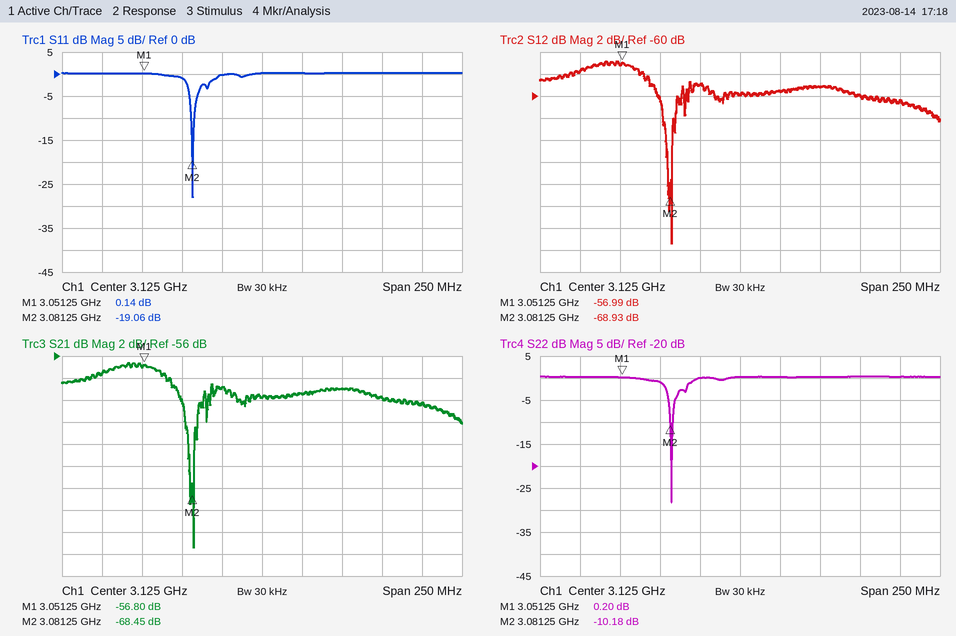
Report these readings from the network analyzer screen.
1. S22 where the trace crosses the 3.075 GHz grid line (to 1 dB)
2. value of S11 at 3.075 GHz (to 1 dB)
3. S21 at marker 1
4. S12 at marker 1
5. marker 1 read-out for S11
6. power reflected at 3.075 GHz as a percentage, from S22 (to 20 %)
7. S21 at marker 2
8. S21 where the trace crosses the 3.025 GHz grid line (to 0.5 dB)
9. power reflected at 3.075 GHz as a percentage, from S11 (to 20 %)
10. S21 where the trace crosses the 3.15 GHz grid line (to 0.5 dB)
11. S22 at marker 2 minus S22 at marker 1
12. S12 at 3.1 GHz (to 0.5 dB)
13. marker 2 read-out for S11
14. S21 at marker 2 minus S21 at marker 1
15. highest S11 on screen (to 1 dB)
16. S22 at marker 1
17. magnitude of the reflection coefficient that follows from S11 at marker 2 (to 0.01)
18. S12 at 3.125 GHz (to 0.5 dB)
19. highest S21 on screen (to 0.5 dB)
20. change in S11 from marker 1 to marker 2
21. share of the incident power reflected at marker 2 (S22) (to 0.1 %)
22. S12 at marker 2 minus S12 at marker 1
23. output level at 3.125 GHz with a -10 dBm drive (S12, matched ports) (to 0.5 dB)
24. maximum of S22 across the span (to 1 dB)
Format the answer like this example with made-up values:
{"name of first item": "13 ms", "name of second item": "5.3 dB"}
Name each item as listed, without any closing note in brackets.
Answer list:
{"S22 where the trace crosses the 3.075 GHz grid line": "-1 dB", "value of S11 at 3.075 GHz": "-1 dB", "S21 at marker 1": "-56.80 dB", "S12 at marker 1": "-56.99 dB", "marker 1 read-out for S11": "0.14 dB", "power reflected at 3.075 GHz as a percentage, from S22": "80 %", "S21 at marker 2": "-68.45 dB", "S21 where the trace crosses the 3.025 GHz grid line": "-57.5 dB", "power reflected at 3.075 GHz as a percentage, from S11": "80 %", "S21 where the trace crosses the 3.15 GHz grid line": "-59.5 dB", "S22 at marker 2 minus S22 at marker 1": "-10.38 dB", "S12 at 3.1 GHz": "-59.0 dB", "marker 2 read-out for S11": "-19.06 dB", "S21 at marker 2 minus S21 at marker 1": "-11.65 dB", "highest S11 on screen": "0 dB", "S22 at marker 1": "0.20 dB", "magnitude of the reflection coefficient that follows from S11 at marker 2": "0.11", "S12 at 3.125 GHz": "-60.0 dB", "highest S21 on screen": "-56.5 dB", "change in S11 from marker 1 to marker 2": "-19.20 dB", "share of the incident power reflected at marker 2 (S22)": "9.6 %", "S12 at marker 2 minus S12 at marker 1": "-11.94 dB", "output level at 3.125 GHz with a -10 dBm drive (S12, matched ports)": "-70.0 dBm", "maximum of S22 across the span": "0 dB"}
